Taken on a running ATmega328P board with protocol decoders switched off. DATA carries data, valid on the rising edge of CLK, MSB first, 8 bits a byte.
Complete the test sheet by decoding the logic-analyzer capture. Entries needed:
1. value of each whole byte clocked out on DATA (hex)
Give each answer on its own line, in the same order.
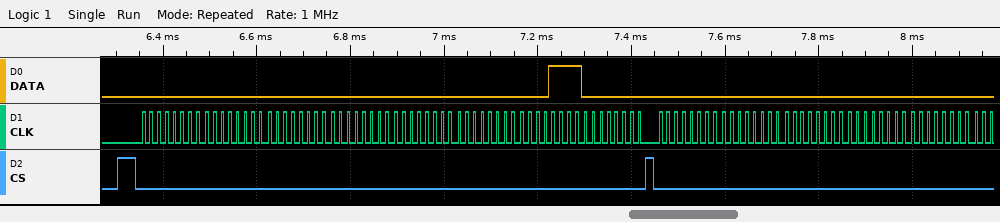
00 00 00 00 00 00 0F 00 00 00 00 00 00
